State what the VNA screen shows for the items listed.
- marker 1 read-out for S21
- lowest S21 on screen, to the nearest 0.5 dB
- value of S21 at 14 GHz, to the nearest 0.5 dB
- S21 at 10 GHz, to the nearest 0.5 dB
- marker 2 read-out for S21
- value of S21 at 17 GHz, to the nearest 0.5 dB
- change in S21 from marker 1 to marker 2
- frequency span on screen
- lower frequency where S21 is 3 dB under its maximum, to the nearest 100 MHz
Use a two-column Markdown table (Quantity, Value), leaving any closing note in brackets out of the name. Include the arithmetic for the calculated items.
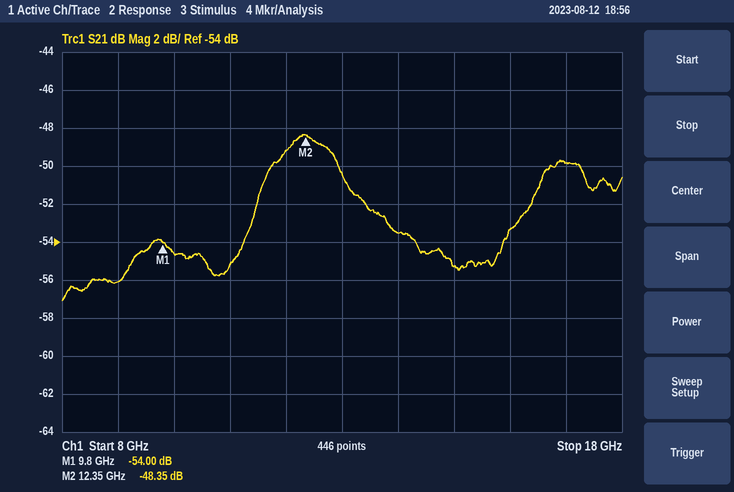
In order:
| Quantity | Value |
|---|---|
| marker 1 read-out for S21 | -54.00 dB |
| lowest S21 on screen, to the nearest 0.5 dB | -57.0 dB |
| value of S21 at 14 GHz, to the nearest 0.5 dB | -53.5 dB |
| S21 at 10 GHz, to the nearest 0.5 dB | -54.5 dB |
| marker 2 read-out for S21 | -48.35 dB |
| value of S21 at 17 GHz, to the nearest 0.5 dB | -50.0 dB |
| change in S21 from marker 1 to marker 2 | -48.35 − (-54) = 5.65 dB |
| frequency span on screen | 10 GHz |
| lower frequency where S21 is 3 dB under its maximum, to the nearest 100 MHz | 11.5 GHz |
